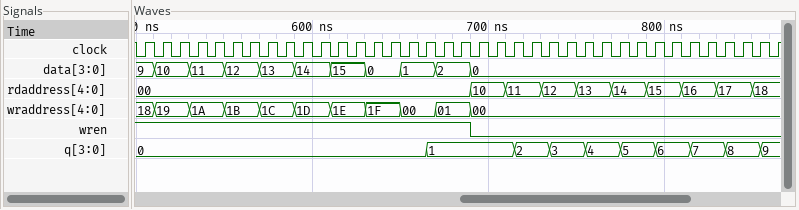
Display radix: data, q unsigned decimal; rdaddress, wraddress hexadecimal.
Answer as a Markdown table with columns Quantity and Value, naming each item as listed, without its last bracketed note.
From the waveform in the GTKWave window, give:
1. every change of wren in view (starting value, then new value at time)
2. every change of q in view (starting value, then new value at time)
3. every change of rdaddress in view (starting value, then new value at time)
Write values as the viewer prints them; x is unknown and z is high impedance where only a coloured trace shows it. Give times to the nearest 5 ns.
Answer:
| Quantity | Value |
|---|---|
| every change of wren in view | 1, 0 at 690 ns |
| every change of q in view | 0, 1 at 665 ns, 2 at 715 ns, 3 at 735 ns, 4 at 755 ns, 5 at 775 ns, 6 at 795 ns, 7 at 815 ns, 8 at 835 ns, 9 at 855 ns |
| every change of rdaddress in view | 00, 10 at 690 ns, 11 at 710 ns, 12 at 730 ns, 13 at 750 ns, 14 at 770 ns, 15 at 790 ns, 16 at 810 ns, 17 at 830 ns, 18 at 850 ns |
